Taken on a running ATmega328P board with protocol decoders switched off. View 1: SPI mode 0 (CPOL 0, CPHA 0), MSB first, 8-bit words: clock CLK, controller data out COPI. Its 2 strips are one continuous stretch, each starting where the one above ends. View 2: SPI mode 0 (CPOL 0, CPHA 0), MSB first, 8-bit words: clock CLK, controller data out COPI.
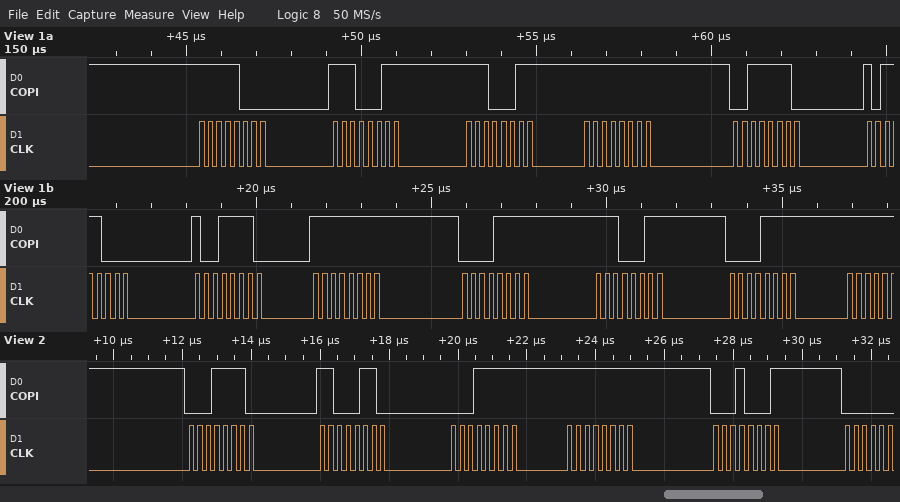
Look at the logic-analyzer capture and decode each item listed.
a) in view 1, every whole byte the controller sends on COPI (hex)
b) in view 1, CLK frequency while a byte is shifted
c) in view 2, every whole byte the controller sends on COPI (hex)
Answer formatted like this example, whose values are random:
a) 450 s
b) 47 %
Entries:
a) F8 E3 E3 FF 3E B8 9E FF 0F E3 0F
b) 4 MHz
c) 1E C6 1F FF 11
